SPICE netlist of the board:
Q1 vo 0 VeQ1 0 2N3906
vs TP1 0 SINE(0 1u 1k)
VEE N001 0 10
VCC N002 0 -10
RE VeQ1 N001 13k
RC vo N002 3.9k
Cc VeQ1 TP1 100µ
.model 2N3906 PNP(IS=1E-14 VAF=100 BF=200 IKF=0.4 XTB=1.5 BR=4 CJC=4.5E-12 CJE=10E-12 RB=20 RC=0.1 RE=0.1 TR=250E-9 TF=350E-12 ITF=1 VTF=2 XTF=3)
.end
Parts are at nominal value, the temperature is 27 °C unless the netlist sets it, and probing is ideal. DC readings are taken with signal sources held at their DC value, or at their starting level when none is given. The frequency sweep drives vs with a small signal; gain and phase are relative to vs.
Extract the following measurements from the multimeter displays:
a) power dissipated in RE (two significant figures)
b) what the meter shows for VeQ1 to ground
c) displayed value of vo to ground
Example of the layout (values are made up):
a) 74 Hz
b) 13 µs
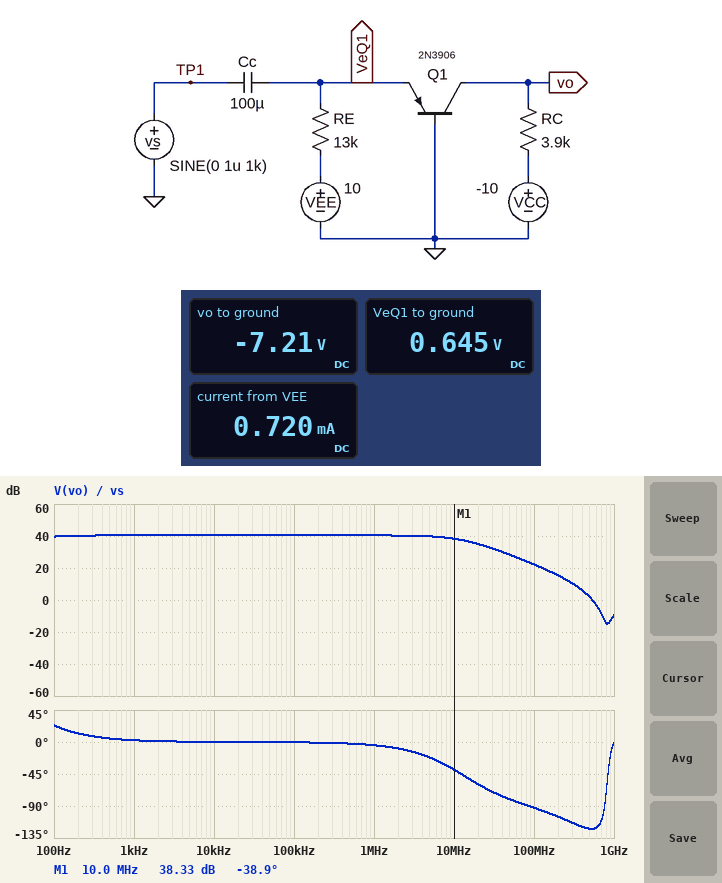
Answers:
a) 6.7 mW
b) 0.645 V
c) -7.21 V
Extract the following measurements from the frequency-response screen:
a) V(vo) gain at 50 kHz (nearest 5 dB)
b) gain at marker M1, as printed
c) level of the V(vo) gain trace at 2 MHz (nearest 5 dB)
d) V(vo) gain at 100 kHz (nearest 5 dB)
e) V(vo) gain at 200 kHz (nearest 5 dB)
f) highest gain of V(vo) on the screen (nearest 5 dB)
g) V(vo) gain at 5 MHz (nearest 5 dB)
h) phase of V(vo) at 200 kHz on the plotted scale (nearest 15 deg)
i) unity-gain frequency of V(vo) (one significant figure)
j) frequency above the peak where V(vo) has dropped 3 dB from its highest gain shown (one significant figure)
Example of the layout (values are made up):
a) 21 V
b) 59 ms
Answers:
a) 40 dB
b) 38.33 dB
c) 40 dB
d) 40 dB
e) 40 dB
f) 40 dB
g) 40 dB
h) 0 deg
i) 500 MHz
j) 10 MHz
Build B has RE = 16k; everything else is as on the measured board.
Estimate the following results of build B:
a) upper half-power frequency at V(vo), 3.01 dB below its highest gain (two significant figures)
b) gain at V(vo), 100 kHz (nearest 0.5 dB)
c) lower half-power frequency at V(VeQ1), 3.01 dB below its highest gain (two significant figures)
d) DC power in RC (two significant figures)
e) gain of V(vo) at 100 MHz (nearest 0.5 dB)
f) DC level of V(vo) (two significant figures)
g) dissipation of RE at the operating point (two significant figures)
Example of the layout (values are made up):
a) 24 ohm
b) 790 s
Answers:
a) 14 MHz
b) 38.5 dB
c) 35 Hz
d) 1.3 mW
e) 21.0 dB
f) -7.7 V
g) 5.5 mW
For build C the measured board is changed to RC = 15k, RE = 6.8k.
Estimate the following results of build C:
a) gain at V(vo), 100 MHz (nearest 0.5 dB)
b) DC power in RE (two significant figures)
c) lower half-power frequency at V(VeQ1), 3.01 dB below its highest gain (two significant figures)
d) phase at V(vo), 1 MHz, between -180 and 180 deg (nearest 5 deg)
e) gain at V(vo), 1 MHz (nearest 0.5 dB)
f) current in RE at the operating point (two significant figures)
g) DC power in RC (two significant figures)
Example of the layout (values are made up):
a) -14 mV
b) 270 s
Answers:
a) -2.5 dB
b) 13 mW
c) 31 Hz
d) -10 deg
e) -2.0 dB
f) 1.4 mA
g) 7.6 mW
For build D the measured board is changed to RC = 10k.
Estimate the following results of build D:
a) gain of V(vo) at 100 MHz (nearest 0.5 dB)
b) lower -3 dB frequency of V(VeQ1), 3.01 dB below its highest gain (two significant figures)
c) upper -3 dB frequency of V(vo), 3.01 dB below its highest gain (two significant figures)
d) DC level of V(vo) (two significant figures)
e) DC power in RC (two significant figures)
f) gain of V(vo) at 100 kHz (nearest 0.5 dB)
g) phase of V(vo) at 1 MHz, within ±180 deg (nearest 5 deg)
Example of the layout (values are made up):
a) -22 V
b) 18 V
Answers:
a) 20.0 dB
b) 41 Hz
c) 4.1 MHz
d) -2.8 V
e) 5.1 mW
f) 48.0 dB
g) -15 deg
